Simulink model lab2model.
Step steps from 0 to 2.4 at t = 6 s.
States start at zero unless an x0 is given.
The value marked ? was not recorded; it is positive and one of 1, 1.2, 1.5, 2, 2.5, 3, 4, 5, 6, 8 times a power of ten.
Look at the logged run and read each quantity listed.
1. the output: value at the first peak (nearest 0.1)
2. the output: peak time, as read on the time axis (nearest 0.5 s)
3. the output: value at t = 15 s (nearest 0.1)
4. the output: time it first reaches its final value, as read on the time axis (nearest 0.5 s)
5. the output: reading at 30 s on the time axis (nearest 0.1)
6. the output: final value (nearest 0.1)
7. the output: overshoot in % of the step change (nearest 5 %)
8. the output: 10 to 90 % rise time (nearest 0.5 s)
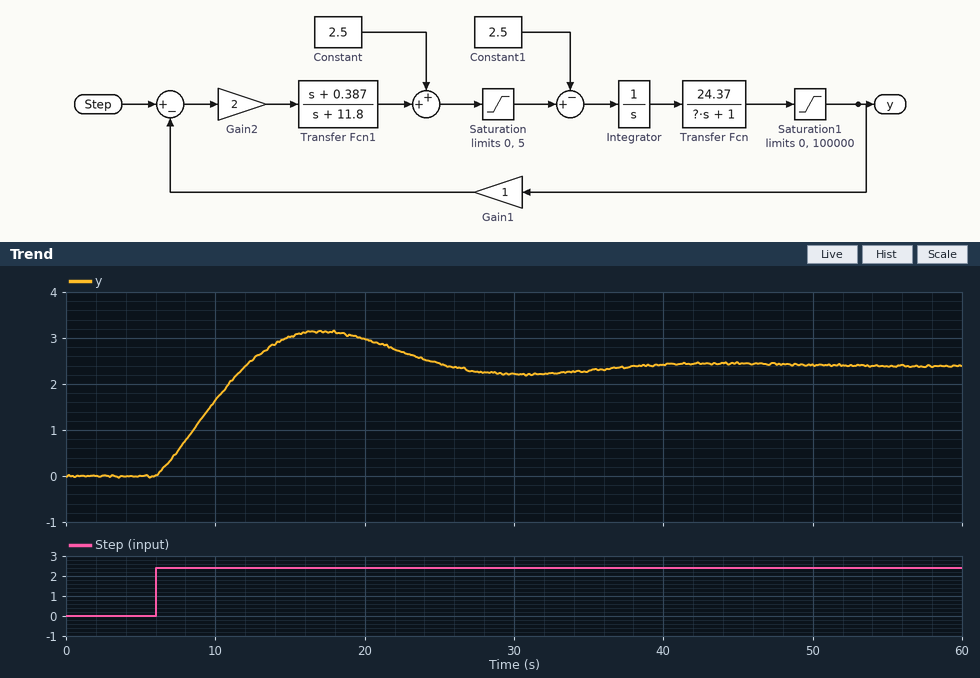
3.1
17.0 s
3.0
12.0 s
2.2
2.4
30 %
4.5 s
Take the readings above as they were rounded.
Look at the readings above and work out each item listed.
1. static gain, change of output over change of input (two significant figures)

1.0
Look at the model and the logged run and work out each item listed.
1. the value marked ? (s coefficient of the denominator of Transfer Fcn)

25
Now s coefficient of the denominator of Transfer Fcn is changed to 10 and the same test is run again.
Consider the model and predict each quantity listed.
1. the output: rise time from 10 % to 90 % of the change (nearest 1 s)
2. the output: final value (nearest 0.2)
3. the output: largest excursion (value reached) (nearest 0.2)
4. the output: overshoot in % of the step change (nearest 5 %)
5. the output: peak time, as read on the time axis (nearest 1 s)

3 s
2.4
2.8
15 %
13 s
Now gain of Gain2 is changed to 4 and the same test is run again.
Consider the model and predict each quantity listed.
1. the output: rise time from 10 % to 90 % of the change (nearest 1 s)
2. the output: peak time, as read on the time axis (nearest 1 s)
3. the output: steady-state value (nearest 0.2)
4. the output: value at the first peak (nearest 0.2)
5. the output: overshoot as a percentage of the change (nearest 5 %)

4 s
14 s
2.4
2.8
20 %
